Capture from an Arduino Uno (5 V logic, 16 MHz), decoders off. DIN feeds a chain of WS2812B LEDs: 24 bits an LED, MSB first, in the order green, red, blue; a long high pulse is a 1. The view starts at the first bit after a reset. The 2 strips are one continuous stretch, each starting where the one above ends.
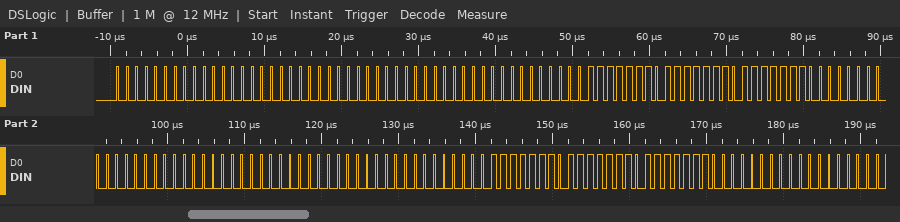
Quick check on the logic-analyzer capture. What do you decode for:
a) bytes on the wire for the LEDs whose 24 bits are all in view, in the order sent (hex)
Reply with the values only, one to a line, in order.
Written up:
00 00 00 00 00 00 7F 7F 7F 00 00 00 00 00 00 7F 7F 7F
